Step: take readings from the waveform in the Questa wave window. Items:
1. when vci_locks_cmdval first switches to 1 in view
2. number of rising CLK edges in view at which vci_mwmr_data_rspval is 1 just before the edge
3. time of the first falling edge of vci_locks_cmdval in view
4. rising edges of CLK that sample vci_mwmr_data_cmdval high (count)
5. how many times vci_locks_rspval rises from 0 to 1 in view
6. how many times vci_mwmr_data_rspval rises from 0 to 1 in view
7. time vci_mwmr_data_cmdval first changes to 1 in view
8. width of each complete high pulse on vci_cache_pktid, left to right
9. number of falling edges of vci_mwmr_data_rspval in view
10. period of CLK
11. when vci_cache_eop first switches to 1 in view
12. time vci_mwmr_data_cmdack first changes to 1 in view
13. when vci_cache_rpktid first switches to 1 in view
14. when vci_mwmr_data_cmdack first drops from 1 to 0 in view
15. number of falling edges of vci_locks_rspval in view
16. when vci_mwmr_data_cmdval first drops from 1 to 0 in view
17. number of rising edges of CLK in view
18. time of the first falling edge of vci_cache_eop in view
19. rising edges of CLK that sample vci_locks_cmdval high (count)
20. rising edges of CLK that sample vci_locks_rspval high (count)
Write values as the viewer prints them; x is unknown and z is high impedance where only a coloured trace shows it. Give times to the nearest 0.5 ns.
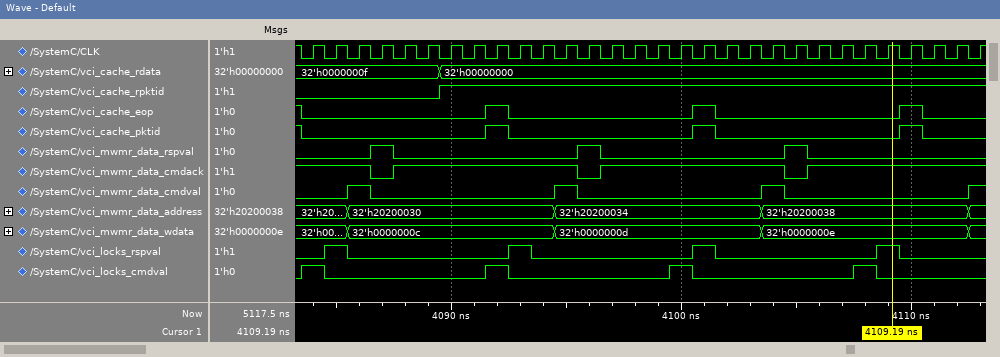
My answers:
4083.5 ns
3
4084.5 ns
4
4
3
4085.5 ns
1 ns, 1 ns, 1 ns
3
1 ns
4091.5 ns
4087.5 ns
4089.5 ns
4086.5 ns
4
4086.5 ns
30
4083.5 ns
4
4
